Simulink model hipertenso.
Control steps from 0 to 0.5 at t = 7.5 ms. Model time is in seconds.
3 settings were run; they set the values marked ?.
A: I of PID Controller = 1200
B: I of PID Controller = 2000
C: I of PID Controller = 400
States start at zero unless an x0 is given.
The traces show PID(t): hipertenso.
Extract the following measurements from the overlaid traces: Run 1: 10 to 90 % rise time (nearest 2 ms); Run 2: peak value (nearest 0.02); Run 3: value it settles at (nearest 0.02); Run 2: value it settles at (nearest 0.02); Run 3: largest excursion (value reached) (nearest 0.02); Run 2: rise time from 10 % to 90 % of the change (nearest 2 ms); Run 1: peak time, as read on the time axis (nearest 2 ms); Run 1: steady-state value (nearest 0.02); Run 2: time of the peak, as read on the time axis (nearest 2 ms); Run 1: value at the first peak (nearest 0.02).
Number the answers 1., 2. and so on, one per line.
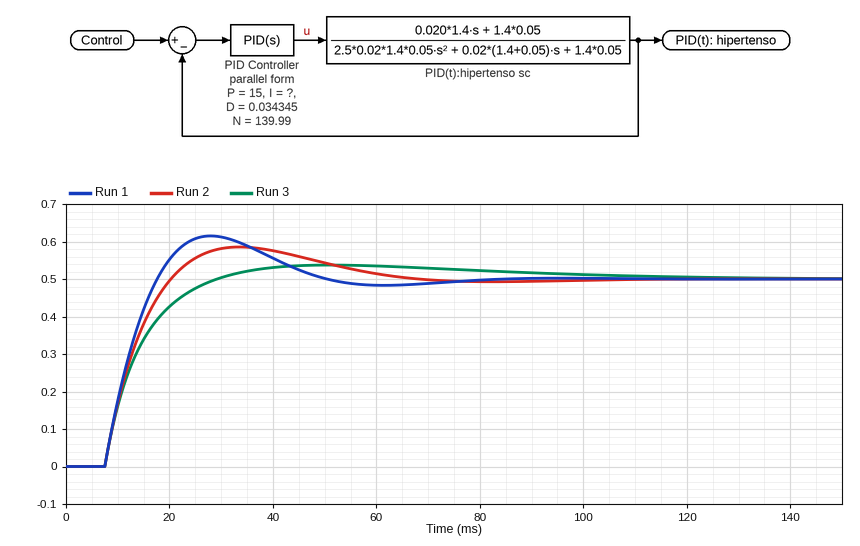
1. 8 ms
2. 0.58
3. 0.50
4. 0.50
5. 0.54
6. 10 ms
7. 28 ms
8. 0.50
9. 34 ms
10. 0.62
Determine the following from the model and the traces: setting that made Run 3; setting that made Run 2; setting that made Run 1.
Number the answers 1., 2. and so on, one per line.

1. C
2. A
3. B
